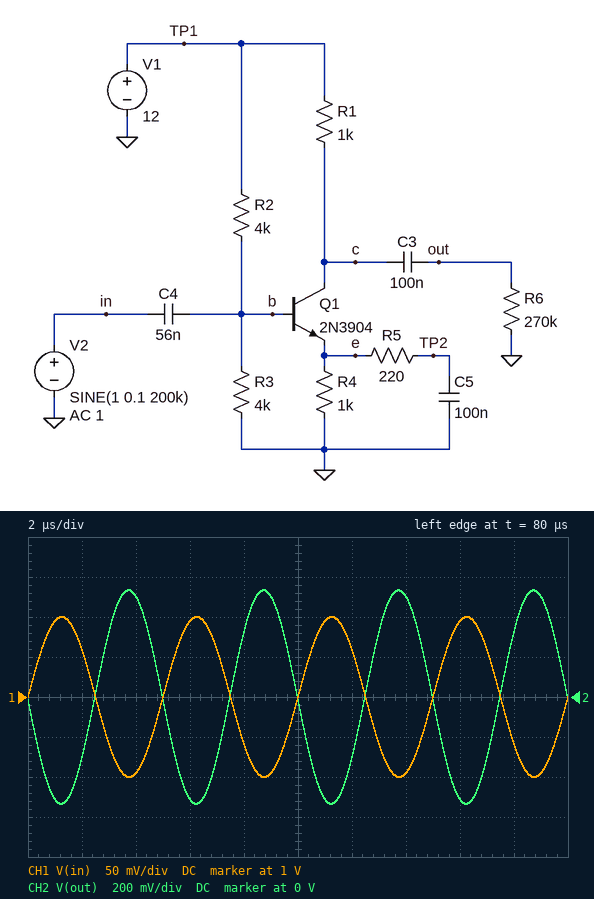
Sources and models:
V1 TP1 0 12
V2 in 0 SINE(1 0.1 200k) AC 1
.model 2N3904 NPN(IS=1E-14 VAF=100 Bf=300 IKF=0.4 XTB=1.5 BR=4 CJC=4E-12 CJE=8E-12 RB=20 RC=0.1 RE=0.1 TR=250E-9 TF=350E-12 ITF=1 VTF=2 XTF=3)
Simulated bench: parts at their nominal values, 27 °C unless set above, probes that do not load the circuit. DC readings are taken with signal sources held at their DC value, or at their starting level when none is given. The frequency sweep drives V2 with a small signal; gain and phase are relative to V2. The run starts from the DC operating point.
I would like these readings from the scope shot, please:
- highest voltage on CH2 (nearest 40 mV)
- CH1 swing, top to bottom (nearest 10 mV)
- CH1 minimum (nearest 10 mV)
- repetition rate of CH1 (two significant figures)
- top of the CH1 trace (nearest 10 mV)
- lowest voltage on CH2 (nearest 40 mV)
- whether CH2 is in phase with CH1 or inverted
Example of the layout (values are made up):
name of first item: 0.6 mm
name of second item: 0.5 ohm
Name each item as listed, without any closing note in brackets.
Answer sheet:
highest voltage on CH2: 520 mV
CH1 swing, top to bottom: 200 mV
CH1 minimum: 900 mV
repetition rate of CH1: 200 kHz
top of the CH1 trace: 1.10 V
lowest voltage on CH2: -520 mV
whether CH2 is in phase with CH1 or inverted: inverted
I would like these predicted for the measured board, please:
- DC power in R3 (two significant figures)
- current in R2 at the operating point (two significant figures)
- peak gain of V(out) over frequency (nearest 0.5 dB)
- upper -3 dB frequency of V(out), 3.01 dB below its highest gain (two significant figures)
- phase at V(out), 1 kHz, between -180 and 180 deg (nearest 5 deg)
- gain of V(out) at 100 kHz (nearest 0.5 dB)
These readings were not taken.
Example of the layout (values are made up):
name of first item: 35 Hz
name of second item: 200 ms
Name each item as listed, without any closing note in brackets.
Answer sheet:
DC power in R3: 8.9 mW
current in R2 at the operating point: 1.5 mA
peak gain of V(out) over frequency: 14.5 dB
upper -3 dB frequency of V(out), 3.01 dB below its highest gain: 47 MHz
phase at V(out), 1 kHz, between -180 and 180 deg: -95 deg
gain of V(out) at 100 kHz: 14.5 dB
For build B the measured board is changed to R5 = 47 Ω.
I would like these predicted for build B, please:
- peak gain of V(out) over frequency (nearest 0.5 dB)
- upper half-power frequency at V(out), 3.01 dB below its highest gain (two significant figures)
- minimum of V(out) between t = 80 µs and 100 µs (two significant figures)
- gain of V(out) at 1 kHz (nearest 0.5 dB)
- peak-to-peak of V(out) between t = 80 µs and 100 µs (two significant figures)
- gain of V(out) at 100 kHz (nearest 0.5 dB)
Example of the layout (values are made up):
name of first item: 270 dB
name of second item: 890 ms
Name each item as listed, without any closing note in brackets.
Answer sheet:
peak gain of V(out) over frequency: 26.0 dB
upper half-power frequency at V(out), 3.01 dB below its highest gain: 35 MHz
minimum of V(out) between t = 80 µs and 100 µs: -1.4 V
gain of V(out) at 1 kHz: -3.5 dB
peak-to-peak of V(out) between t = 80 µs and 100 µs: 3.3 V
gain of V(out) at 100 kHz: 25.5 dB
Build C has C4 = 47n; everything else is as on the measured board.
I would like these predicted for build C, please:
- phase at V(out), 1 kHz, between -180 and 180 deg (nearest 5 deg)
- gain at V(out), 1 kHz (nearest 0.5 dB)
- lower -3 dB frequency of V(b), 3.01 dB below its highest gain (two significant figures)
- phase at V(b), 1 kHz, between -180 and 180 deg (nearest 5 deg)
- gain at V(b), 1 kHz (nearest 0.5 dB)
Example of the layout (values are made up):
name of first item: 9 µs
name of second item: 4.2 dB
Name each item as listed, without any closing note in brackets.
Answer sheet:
phase at V(out), 1 kHz, between -180 and 180 deg: -90 deg
gain at V(out), 1 kHz: -4.0 dB
lower -3 dB frequency of V(b), 3.01 dB below its highest gain: 1.7 kHz
phase at V(b), 1 kHz, between -180 and 180 deg: 60 deg
gain at V(b), 1 kHz: -6.0 dB
